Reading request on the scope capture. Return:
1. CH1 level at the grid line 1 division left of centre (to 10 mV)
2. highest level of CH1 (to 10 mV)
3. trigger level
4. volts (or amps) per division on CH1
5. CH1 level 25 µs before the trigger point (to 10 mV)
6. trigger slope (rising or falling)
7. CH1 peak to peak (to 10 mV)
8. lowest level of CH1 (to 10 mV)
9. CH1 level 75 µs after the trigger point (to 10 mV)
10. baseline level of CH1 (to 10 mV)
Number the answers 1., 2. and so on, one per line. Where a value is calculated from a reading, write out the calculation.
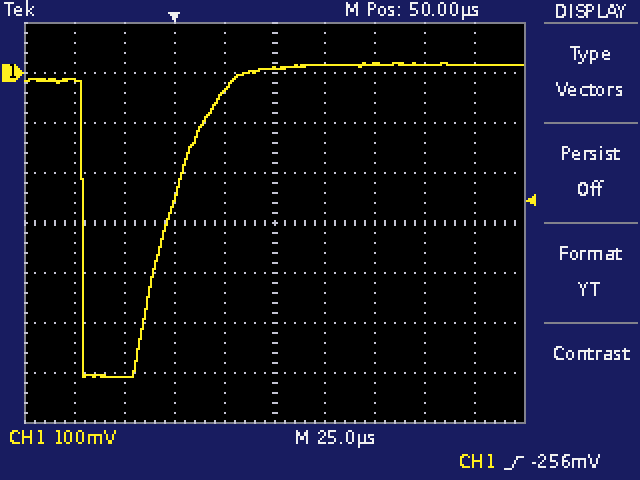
1. -40 mV
2. 20 mV
3. -256 mV
4. 100 mV
5. -610 mV
6. rising
7. 20 mV − (-610 mV) = 630 mV
8. -610 mV
9. 20 mV
10. 20 mV
